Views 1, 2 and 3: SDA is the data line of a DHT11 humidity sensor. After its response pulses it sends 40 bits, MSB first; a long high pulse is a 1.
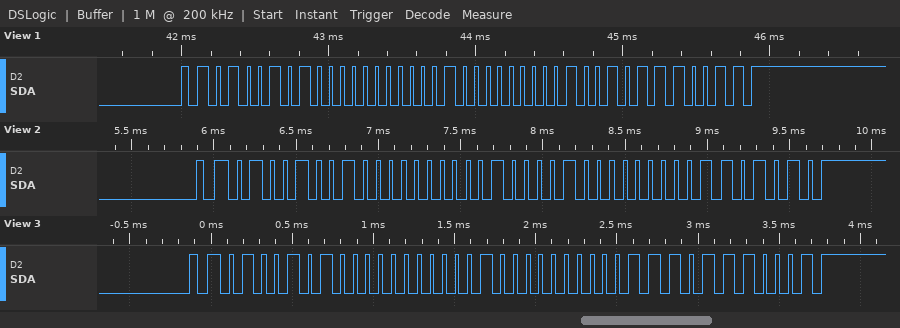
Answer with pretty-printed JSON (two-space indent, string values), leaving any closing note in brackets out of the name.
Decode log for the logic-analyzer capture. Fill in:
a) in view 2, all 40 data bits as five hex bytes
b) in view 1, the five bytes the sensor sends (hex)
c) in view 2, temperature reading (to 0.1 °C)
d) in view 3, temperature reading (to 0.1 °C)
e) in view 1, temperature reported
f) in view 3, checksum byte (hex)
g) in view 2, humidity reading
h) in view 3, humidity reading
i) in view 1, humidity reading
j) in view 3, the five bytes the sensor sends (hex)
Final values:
{
  "in view 2, all 40 data bits as five hex bytes": "49 00 21 00 6A",
  "in view 1, the five bytes the sensor sends": "4A 00 20 09 73",
  "in view 2, temperature reading": "33.0 °C",
  "in view 3, temperature reading": "32.7 °C",
  "in view 1, temperature reported": "32.9 °C",
  "in view 3, checksum byte": "0x71",
  "in view 2, humidity reading": "73 %",
  "in view 3, humidity reading": "74 %",
  "in view 1, humidity reading": "74 %",
  "in view 3, the five bytes the sensor sends": "4A 00 20 07 71"
}
